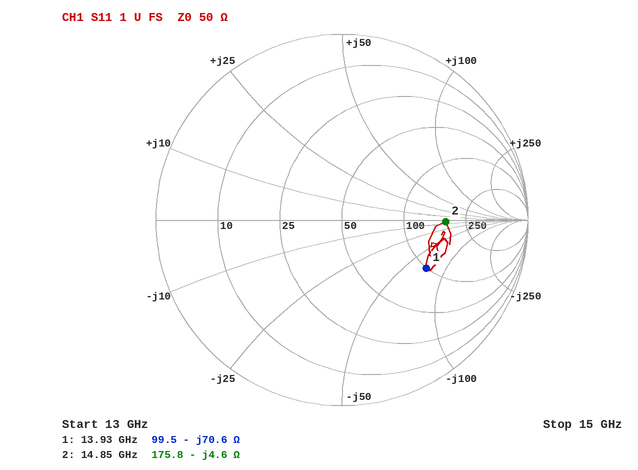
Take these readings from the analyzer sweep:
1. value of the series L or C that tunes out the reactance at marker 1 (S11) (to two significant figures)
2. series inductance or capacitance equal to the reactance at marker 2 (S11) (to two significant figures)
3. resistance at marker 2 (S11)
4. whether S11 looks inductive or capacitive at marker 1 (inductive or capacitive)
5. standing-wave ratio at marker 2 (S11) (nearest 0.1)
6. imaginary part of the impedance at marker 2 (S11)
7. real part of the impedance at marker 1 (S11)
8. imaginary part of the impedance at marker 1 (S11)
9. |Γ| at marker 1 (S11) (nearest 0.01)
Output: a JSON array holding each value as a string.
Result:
["810 pH", "2.3 pF", "175.8 Ω", "capacitive", "3.5", "-4.6 Ω", "99.5 Ω", "-70.6 Ω", "0.52"]
